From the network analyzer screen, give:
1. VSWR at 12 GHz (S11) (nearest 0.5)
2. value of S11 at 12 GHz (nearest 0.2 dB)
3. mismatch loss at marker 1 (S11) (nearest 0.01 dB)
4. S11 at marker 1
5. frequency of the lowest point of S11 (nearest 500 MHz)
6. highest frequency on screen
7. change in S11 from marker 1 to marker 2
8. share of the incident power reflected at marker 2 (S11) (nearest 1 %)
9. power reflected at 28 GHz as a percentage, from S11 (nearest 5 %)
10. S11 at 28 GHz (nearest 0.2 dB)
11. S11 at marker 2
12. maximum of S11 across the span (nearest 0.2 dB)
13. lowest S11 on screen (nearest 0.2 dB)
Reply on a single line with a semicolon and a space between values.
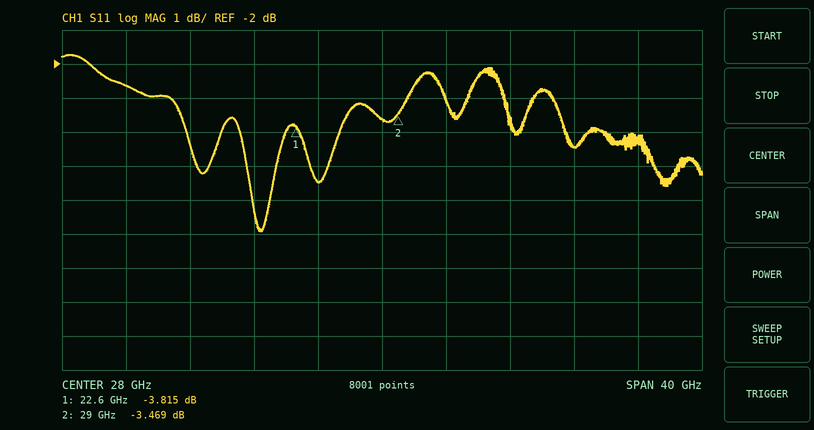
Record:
6.5; -2.6 dB; 2.33 dB; -3.815 dB; 20.5 GHz; 48 GHz; 0.346 dB; 45 %; 45 %; -3.6 dB; -3.469 dB; -1.8 dB; -7.0 dB
